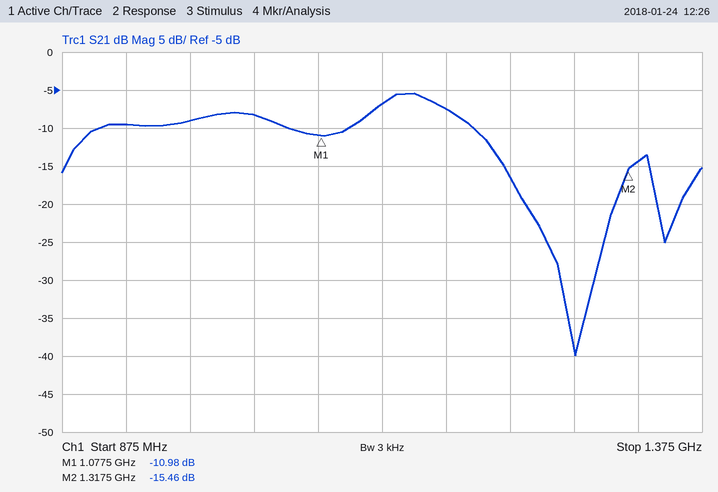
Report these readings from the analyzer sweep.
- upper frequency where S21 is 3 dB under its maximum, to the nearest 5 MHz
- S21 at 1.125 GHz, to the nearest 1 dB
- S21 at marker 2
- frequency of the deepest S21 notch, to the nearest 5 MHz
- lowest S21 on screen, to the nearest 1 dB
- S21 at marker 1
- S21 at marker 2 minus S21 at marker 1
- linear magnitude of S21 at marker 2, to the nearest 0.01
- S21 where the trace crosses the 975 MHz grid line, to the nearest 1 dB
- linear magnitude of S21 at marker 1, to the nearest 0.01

1.185 GHz
-7 dB
-15.46 dB
1.275 GHz
-40 dB
-10.98 dB
-4.48 dB
0.17
-9 dB
0.28
